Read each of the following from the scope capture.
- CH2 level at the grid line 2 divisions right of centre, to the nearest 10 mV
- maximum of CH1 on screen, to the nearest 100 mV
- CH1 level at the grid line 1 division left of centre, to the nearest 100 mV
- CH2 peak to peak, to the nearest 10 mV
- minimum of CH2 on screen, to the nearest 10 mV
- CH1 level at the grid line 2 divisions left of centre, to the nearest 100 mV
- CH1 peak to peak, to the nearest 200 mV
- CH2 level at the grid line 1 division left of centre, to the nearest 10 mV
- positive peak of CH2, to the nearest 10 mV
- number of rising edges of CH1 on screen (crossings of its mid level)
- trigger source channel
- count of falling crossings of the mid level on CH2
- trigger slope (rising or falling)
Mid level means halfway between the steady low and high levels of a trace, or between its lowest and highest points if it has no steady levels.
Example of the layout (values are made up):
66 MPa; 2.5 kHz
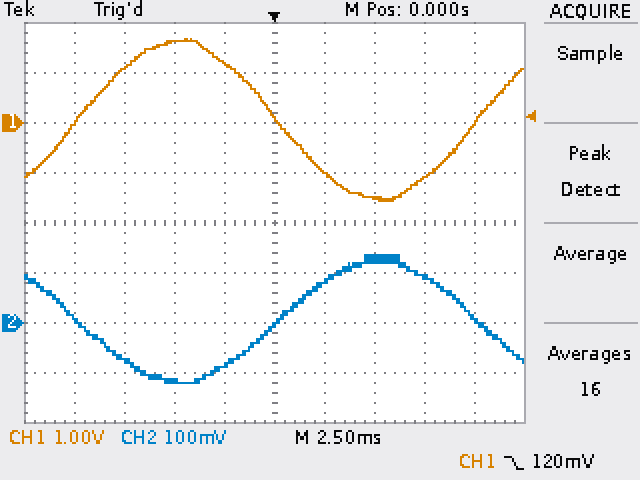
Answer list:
130 mV; 1.7 V; 1.2 V; 260 mV; -120 mV; 1.6 V; 3.2 V; -80 mV; 140 mV; 2; CH1; 2; falling
